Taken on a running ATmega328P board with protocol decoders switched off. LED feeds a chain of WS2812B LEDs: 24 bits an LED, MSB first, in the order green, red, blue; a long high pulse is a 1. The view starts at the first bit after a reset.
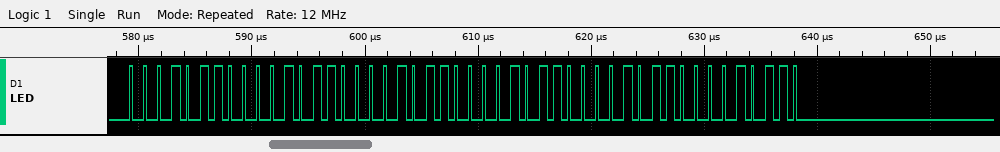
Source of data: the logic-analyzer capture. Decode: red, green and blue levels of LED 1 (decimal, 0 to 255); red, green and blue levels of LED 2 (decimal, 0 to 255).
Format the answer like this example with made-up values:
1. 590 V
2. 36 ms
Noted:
1. 22, 22, 22
2. 22, 22, 22
